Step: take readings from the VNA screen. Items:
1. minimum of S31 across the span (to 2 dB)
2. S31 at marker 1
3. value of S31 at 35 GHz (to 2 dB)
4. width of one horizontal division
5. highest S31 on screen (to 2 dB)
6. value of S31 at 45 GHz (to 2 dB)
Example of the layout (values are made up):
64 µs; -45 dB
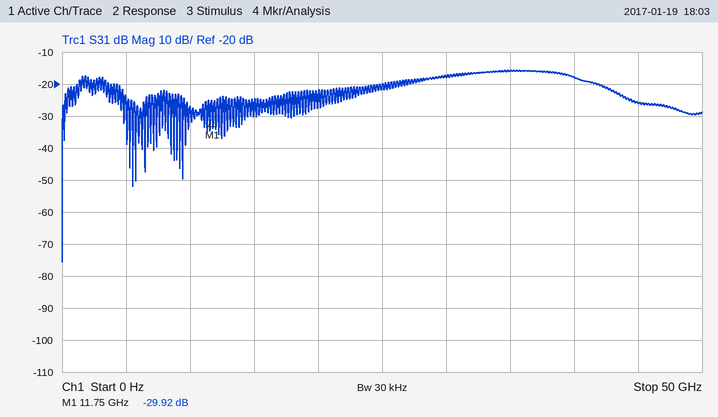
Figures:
-76 dB; -29.92 dB; -16 dB; 5 GHz; -16 dB; -26 dB
